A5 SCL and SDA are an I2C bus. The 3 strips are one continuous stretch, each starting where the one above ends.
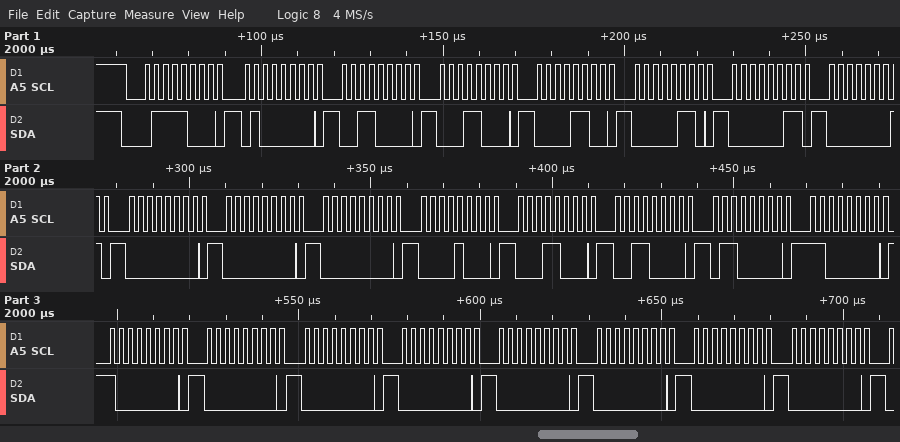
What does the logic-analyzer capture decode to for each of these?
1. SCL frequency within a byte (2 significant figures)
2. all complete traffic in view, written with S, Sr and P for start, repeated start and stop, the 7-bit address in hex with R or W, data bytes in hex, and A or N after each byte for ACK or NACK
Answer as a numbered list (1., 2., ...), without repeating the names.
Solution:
1. 400 kHz
2. S 3CW A 40 A 30 A 18 A 0C A 06 A 03 A 01 A 00 A 00 A 00 A 08 A 18 A 30 A 60 A C0 A 80 A 00 A 00 A 00 A 00 A 00 A 00 A 00 A
